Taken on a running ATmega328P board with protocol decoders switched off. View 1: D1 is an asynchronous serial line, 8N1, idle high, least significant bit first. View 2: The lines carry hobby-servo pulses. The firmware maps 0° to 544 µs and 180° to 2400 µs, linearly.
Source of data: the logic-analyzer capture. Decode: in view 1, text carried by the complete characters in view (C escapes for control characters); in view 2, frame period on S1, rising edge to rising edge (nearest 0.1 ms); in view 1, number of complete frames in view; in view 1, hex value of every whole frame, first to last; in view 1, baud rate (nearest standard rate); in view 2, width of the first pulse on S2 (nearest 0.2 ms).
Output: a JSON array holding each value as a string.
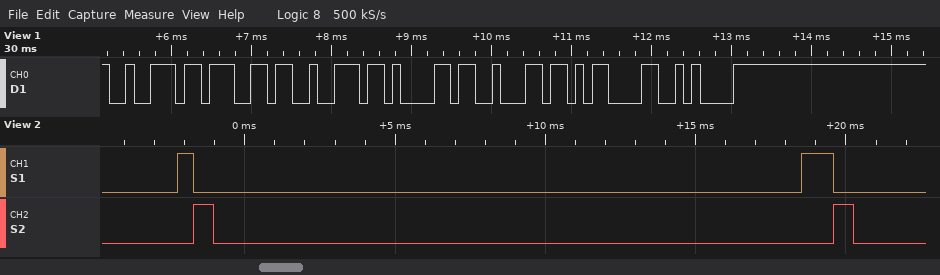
["\"rgrab\\r\\n\"", "20.8 ms", "7", "0x72 0x67 0x72 0x61 0x62 0x0D 0x0A", "9600 baud", "0.6 ms"]
